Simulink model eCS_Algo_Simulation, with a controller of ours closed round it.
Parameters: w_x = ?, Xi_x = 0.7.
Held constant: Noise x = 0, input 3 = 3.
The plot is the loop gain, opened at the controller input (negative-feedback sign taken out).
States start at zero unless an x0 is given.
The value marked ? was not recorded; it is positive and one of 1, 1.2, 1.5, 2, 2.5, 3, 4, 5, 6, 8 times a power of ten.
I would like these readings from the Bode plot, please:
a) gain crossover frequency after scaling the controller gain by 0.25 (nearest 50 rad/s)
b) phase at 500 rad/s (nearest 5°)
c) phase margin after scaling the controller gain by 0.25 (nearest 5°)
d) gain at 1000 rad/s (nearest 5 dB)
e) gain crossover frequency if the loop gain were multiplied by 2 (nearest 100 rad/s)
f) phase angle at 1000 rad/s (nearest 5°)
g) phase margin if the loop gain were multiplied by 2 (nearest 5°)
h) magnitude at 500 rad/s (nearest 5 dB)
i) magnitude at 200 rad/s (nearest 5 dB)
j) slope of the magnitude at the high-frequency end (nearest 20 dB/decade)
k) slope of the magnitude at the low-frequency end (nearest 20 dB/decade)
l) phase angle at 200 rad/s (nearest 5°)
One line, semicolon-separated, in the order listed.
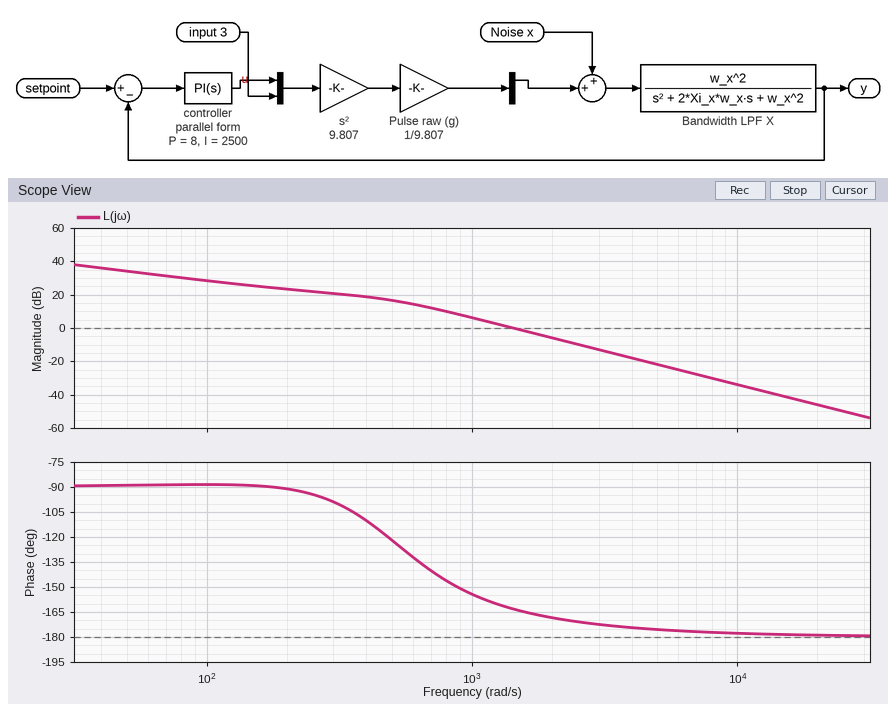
700 rad/s; -120°; 40°; 5 dB; 2000 rad/s; -155°; 10°; 15 dB; 25 dB; -40 dB/decade; -20 dB/decade; -90°
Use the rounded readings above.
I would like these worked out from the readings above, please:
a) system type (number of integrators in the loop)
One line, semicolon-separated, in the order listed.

1
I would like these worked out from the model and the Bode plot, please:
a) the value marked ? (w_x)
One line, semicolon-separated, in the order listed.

500
